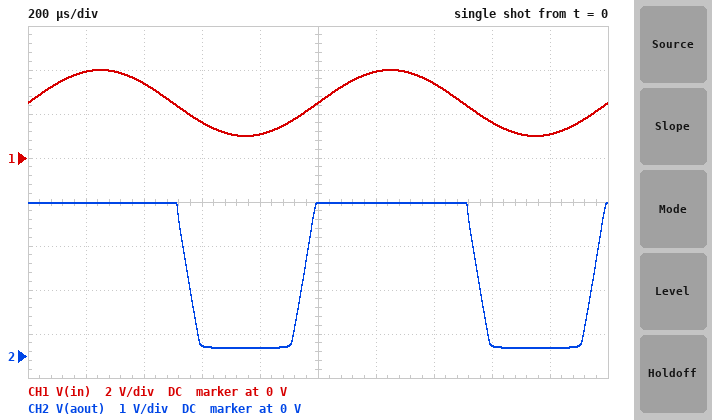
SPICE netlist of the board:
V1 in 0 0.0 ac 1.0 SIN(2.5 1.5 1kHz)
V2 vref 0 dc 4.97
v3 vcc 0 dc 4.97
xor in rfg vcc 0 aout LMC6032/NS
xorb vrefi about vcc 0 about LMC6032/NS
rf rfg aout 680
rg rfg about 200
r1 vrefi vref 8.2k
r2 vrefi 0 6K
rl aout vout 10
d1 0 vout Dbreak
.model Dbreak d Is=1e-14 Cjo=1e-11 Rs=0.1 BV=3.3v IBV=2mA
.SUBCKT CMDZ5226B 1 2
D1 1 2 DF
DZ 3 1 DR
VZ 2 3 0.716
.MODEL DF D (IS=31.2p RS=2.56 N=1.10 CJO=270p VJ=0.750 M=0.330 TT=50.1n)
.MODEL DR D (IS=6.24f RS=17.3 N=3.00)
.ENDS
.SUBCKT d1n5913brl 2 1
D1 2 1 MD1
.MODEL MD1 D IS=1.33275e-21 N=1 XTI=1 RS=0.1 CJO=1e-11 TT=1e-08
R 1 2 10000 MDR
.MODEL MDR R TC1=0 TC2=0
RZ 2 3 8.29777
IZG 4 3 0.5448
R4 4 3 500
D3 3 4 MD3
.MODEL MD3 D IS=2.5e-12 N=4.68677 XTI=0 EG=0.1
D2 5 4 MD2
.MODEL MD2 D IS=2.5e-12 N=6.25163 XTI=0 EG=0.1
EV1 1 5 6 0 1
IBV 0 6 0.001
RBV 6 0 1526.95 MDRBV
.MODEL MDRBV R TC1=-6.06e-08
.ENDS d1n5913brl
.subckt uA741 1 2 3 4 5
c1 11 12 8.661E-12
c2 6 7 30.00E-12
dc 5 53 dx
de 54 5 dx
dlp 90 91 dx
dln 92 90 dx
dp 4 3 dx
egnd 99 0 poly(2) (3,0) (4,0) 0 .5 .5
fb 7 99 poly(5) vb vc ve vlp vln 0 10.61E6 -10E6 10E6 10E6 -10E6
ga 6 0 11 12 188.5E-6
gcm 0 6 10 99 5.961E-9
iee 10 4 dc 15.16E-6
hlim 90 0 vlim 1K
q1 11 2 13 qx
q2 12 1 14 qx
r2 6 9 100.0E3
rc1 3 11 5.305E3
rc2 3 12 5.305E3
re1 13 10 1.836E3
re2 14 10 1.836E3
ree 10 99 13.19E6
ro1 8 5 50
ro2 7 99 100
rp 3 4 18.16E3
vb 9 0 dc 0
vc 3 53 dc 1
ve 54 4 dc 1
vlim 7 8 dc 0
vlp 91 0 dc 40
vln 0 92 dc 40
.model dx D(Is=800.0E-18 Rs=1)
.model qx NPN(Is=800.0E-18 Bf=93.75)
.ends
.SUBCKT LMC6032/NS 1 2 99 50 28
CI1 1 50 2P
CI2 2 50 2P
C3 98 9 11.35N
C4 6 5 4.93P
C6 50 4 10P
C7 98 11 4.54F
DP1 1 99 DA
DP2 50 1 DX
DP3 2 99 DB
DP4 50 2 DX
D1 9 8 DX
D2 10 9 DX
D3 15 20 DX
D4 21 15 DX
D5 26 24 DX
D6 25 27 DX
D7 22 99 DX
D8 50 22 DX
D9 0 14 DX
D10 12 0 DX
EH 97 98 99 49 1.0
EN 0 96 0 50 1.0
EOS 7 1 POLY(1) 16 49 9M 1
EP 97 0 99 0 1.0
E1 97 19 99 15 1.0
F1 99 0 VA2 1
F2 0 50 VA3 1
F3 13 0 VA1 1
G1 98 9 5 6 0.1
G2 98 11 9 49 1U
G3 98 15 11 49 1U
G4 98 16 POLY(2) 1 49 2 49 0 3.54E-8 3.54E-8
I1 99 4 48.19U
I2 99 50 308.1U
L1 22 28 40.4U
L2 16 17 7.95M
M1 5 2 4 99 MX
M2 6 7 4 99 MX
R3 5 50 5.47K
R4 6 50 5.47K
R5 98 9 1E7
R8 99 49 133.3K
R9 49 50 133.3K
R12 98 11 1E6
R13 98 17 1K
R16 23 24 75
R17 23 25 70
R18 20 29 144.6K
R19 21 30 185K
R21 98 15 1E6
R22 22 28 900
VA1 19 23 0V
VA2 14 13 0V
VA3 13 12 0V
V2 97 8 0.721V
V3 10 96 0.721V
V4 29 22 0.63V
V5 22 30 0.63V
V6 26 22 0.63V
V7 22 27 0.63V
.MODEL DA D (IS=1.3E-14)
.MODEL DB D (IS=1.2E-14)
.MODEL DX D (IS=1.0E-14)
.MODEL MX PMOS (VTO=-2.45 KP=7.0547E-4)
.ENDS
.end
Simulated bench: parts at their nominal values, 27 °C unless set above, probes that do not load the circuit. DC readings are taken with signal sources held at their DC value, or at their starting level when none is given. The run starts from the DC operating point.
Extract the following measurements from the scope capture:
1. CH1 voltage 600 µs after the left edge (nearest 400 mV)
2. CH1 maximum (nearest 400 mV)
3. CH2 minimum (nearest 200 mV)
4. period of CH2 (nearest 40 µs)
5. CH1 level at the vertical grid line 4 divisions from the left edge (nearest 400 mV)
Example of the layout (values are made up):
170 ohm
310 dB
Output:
1.6 V
4.0 V
200 mV
1.00 ms
1.2 V
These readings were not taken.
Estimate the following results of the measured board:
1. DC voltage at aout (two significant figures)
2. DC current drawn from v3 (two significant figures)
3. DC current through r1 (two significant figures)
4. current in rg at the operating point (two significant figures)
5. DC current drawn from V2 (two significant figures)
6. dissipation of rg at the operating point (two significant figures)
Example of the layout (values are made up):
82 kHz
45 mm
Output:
190 mV
2.9 mA
350 µA
2.2 mA
350 µA
950 µW
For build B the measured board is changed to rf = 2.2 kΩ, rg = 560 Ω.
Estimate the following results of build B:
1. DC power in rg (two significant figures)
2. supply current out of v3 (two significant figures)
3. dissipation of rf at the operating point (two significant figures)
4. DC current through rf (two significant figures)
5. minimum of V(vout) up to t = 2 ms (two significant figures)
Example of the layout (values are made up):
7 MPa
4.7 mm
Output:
310 µW
1.5 mA
1.2 mW
740 µA
57 mV
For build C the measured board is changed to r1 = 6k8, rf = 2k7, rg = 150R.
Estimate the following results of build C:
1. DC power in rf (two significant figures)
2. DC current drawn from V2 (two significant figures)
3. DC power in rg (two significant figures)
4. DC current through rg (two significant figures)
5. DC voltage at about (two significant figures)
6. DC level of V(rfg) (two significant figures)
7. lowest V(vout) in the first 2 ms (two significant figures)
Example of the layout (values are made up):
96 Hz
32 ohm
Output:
1.7 mW
390 µA
96 µW
800 µA
2.3 V
2.2 V
62 mV
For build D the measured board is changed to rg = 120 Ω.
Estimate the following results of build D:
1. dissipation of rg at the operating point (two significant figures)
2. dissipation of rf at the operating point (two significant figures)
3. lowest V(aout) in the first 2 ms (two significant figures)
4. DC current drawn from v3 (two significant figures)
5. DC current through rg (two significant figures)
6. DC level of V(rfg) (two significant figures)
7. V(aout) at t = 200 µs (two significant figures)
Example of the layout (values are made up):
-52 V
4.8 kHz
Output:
680 µW
3.8 mW
210 mV
3.1 mA
2.4 mA
1.8 V
3.5 V
